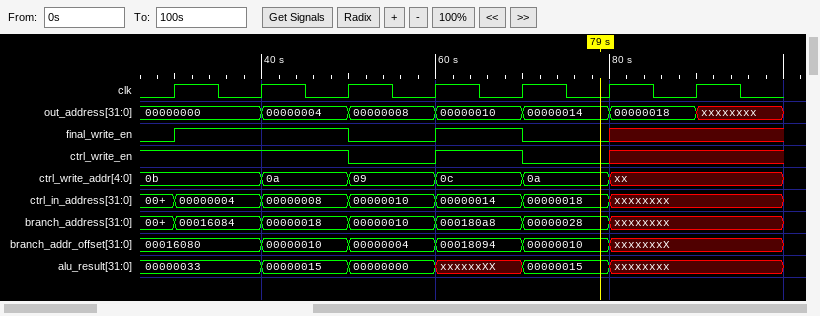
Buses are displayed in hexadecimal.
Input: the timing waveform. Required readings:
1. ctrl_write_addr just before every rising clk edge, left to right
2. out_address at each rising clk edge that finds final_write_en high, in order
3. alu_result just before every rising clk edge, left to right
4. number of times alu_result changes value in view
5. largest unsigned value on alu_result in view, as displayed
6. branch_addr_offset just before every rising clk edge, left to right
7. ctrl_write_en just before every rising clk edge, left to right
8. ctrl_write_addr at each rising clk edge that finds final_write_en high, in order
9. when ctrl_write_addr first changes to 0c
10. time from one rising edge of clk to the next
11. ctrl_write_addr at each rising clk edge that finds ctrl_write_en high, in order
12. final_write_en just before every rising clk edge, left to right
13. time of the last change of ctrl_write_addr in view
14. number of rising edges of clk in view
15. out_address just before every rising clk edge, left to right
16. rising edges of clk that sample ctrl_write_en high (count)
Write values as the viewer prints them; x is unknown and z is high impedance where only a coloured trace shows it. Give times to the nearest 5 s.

0b, 0b, 0a, 09, 0c, 0a, xx
00000000, 00000004, 00000010
00000033, 00000033, 00000015, 00000000, xxxxxxXX, 00000015, xxxxxxxx
5
00000033
00016080, 00016080, 00000010, 00000004, 00018094, 00000010, xxxxxxxX
1 1 1 0 1 0 x
0b, 0a, 0c
60 s
10 s
0b, 0b, 0a, 0c
0 1 1 0 1 0 x
80 s
7
00000000, 00000000, 00000004, 00000008, 00000010, 00000014, 00000018
4
